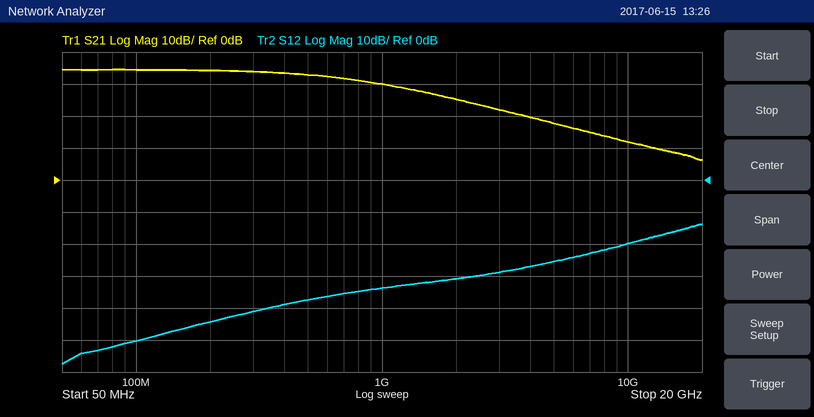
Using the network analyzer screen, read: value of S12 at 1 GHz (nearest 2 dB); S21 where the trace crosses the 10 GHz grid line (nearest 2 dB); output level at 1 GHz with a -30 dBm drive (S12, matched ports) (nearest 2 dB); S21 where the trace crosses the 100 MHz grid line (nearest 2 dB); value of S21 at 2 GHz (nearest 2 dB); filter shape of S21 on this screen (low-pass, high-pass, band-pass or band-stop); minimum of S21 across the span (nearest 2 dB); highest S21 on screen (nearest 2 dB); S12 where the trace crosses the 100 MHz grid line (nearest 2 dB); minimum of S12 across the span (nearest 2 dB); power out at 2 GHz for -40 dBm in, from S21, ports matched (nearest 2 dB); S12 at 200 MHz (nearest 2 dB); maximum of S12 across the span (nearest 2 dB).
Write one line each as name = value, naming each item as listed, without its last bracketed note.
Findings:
value of S12 at 1 GHz = -34 dB
S21 where the trace crosses the 10 GHz grid line = 12 dB
output level at 1 GHz with a -30 dBm drive (S12, matched ports) = -64 dBm
S21 where the trace crosses the 100 MHz grid line = 34 dB
value of S21 at 2 GHz = 26 dB
filter shape of S21 on this screen = low-pass
minimum of S21 across the span = 6 dB
highest S21 on screen = 34 dB
S12 where the trace crosses the 100 MHz grid line = -50 dB
minimum of S12 across the span = -58 dB
power out at 2 GHz for -40 dBm in, from S21, ports matched = -14 dBm
S12 at 200 MHz = -44 dB
maximum of S12 across the span = -14 dB
